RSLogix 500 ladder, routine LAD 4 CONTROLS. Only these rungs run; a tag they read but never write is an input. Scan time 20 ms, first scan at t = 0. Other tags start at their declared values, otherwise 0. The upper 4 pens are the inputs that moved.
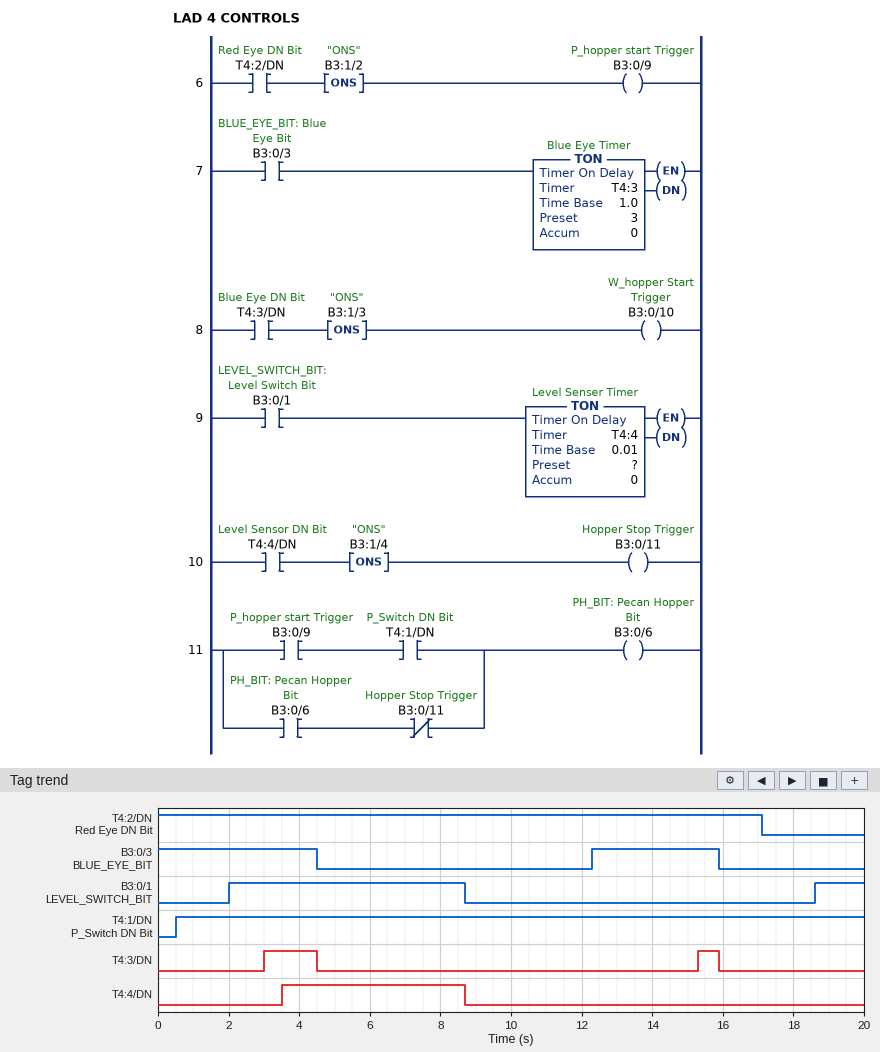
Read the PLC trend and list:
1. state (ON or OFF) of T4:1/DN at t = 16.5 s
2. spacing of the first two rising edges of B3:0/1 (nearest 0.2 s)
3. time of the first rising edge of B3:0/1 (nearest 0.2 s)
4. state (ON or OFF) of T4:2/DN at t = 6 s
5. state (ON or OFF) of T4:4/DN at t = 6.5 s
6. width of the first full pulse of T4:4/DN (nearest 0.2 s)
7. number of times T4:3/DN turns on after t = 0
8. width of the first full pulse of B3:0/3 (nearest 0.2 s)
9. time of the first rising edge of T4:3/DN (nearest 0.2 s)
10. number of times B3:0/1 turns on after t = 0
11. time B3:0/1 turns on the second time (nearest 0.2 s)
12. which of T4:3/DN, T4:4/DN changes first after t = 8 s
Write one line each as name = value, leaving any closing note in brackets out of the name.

state (ON or OFF) of T4:1/DN at t = 16.5 s = ON
spacing of the first two rising edges of B3:0/1 = 16.6 s
time of the first rising edge of B3:0/1 = 2.0 s
state (ON or OFF) of T4:2/DN at t = 6 s = ON
state (ON or OFF) of T4:4/DN at t = 6.5 s = ON
width of the first full pulse of T4:4/DN = 5.2 s
number of times T4:3/DN turns on after t = 0 = 2
width of the first full pulse of B3:0/3 = 3.6 s
time of the first rising edge of T4:3/DN = 3.0 s
number of times B3:0/1 turns on after t = 0 = 2
time B3:0/1 turns on the second time = 18.6 s
which of T4:3/DN, T4:4/DN changes first after t = 8 s = T4:4/DN
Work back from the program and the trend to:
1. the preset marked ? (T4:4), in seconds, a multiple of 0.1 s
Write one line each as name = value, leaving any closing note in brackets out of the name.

the preset marked ? (T4:4), in seconds, a multiple of 0.1 s = 1.5 s
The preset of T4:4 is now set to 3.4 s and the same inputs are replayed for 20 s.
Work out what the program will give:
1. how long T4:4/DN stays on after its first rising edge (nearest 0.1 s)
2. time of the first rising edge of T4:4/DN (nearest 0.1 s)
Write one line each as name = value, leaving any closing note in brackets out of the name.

how long T4:4/DN stays on after its first rising edge = 3.3 s
time of the first rising edge of T4:4/DN = 5.4 s
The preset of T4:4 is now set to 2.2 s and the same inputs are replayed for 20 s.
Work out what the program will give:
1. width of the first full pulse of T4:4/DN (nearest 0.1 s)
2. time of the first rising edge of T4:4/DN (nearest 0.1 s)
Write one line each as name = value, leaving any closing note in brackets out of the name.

width of the first full pulse of T4:4/DN = 4.5 s
time of the first rising edge of T4:4/DN = 4.2 s
